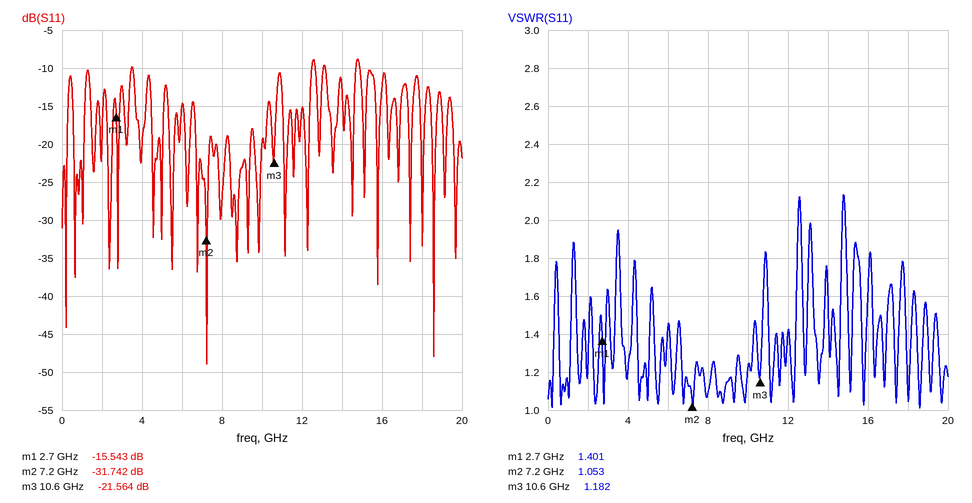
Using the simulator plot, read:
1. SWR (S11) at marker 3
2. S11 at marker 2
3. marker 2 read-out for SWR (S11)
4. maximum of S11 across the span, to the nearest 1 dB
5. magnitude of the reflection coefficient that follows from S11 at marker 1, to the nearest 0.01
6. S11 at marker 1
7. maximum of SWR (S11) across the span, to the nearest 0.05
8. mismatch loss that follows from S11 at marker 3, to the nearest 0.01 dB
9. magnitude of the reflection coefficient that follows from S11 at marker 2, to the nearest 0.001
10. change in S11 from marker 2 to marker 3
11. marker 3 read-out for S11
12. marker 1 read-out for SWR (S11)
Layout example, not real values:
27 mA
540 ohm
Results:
1.182
-31.742 dB
1.053
-9 dB
0.17
-15.543 dB
2.15
0.03 dB
0.026
10.178 dB
-21.564 dB
1.401
